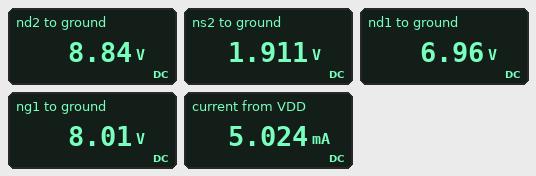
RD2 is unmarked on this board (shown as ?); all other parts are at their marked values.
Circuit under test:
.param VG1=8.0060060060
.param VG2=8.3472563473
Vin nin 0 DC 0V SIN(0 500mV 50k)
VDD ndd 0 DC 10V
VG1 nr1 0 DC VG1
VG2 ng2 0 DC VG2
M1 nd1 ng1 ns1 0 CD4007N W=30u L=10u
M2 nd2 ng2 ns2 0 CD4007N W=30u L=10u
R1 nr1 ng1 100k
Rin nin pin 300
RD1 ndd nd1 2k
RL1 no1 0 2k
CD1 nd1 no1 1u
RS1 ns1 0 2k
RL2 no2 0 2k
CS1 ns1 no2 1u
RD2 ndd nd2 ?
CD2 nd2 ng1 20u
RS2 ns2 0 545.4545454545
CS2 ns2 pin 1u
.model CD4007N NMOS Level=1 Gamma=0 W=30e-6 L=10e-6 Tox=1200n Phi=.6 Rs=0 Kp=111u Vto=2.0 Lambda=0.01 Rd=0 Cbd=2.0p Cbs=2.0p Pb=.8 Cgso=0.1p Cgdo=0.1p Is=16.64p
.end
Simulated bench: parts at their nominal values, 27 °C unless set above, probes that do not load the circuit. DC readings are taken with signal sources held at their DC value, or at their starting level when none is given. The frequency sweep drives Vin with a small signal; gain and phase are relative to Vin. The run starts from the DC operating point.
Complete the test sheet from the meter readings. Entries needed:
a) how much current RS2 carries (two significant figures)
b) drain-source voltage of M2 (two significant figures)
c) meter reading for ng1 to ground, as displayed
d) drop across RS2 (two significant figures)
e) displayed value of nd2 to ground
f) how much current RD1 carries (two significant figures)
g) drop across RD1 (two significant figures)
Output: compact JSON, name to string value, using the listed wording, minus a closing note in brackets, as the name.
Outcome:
{"how much current RS2 carries": "3.5 mA", "drain-source voltage of M2": "6.9 V", "meter reading for ng1 to ground, as displayed": "8.01 V", "drop across RS2": "1.9 V", "displayed value of nd2 to ground": "8.84 V", "how much current RD1 carries": "1.5 mA", "drop across RD1": "3.0 V"}
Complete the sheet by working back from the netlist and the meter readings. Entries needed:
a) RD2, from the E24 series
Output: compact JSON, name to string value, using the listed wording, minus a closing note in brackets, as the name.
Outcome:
{"RD2, from the E24 series": "330 Ω"}
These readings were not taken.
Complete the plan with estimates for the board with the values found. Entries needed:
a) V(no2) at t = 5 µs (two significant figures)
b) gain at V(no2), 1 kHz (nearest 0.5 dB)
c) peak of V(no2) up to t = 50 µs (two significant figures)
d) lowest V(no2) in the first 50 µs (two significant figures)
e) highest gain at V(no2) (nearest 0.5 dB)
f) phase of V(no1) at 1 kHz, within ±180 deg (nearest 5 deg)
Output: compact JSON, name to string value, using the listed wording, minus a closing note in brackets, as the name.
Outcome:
{"V(no2) at t = 5 µs": "63 mV", "gain at V(no2), 1 kHz": "-18.0 dB", "peak of V(no2) up to t = 50 µs": "63 mV", "lowest V(no2) in the first 50 µs": "-66 mV", "highest gain at V(no2)": "-18.0 dB", "phase of V(no1) at 1 kHz, within ±180 deg": "-160 deg"}
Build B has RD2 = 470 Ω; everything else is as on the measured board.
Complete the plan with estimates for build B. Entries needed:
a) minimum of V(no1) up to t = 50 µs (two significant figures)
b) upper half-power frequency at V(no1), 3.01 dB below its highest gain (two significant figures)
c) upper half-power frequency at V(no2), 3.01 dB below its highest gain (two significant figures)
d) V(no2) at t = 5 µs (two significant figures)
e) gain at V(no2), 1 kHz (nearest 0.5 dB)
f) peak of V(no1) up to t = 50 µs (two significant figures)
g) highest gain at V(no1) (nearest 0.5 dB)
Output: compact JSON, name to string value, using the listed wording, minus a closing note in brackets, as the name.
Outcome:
{"minimum of V(no1) up to t = 50 µs": "-89 mV", "upper half-power frequency at V(no1), 3.01 dB below its highest gain": "370 MHz", "upper half-power frequency at V(no2), 3.01 dB below its highest gain": "260 MHz", "V(no2) at t = 5 µs": "89 mV", "gain at V(no2), 1 kHz": "-15.0 dB", "peak of V(no1) up to t = 50 µs": "93 mV", "highest gain at V(no1)": "-14.5 dB"}
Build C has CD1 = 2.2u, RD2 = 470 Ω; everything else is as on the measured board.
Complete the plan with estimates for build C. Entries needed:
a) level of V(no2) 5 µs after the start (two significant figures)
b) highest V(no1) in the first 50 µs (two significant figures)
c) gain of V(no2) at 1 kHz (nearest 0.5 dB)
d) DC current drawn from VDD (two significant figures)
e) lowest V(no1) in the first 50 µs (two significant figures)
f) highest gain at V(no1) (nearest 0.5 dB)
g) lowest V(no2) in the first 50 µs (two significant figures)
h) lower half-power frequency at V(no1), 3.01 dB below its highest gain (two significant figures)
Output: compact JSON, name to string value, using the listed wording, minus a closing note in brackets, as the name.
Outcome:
{"level of V(no2) 5 µs after the start": "89 mV", "highest V(no1) in the first 50 µs": "93 mV", "gain of V(no2) at 1 kHz": "-15.0 dB", "DC current drawn from VDD": "5.0 mA", "lowest V(no1) in the first 50 µs": "-89 mV", "highest gain at V(no1)": "-14.5 dB", "lowest V(no2) in the first 50 µs": "-93 mV", "lower half-power frequency at V(no1), 3.01 dB below its highest gain": "280 Hz"}
